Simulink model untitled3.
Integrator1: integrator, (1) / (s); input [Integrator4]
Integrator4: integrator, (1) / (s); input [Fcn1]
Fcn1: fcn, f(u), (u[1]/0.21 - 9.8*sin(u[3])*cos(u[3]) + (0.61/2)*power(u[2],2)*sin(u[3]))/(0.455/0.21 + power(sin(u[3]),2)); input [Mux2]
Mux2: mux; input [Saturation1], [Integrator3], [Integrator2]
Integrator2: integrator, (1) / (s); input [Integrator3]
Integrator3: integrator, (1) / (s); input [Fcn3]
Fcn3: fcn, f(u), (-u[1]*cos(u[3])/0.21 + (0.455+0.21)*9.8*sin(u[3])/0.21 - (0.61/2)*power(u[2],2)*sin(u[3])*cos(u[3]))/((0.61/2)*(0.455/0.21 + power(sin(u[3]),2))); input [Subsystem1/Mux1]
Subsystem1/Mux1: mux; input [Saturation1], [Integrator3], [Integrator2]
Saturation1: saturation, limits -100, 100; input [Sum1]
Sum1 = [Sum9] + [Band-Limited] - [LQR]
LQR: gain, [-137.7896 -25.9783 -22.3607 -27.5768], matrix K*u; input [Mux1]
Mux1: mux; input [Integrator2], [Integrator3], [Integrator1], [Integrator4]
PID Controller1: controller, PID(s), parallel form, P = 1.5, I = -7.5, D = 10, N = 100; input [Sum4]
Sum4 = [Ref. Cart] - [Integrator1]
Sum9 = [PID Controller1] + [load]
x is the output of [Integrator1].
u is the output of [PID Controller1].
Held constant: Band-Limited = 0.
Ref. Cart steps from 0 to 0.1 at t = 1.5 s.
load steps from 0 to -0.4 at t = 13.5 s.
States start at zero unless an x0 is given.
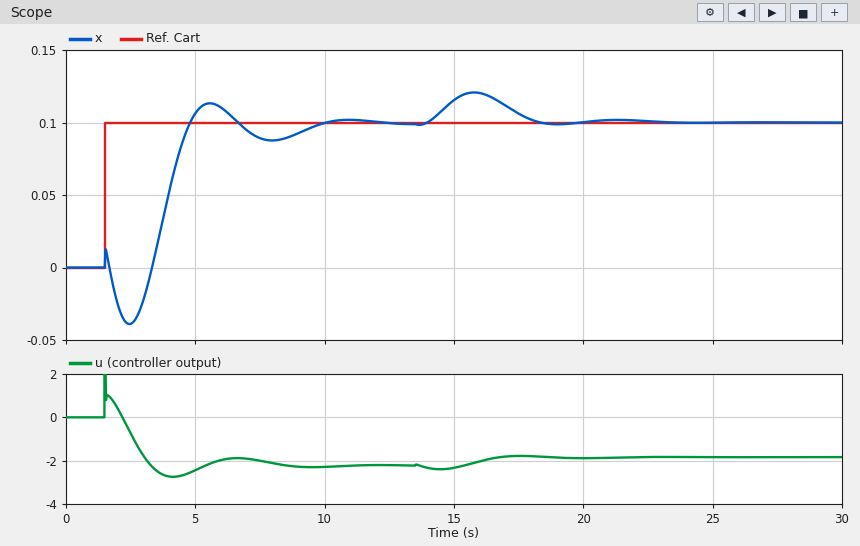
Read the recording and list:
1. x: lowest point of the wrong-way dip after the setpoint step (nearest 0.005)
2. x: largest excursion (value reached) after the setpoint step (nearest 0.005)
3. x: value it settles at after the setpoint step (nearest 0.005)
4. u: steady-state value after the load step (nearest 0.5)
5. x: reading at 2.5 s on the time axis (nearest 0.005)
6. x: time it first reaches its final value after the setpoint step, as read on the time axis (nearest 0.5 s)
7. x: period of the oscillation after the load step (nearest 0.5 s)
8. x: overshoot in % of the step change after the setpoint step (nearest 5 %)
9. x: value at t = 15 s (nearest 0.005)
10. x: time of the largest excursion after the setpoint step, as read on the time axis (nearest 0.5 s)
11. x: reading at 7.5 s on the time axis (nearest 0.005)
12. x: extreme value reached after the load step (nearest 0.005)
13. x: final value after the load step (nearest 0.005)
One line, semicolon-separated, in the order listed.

-0.040; 0.115; 0.100; -2.0; -0.040; 5.0 s; 5.5 s; 15 %; 0.115; 5.5 s; 0.090; 0.120; 0.100
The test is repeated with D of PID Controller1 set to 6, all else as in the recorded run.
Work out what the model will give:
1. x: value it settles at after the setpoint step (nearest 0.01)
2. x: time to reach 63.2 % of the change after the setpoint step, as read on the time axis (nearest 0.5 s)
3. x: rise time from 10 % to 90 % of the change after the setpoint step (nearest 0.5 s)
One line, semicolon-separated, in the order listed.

0.10; 4.5 s; 2.0 s
